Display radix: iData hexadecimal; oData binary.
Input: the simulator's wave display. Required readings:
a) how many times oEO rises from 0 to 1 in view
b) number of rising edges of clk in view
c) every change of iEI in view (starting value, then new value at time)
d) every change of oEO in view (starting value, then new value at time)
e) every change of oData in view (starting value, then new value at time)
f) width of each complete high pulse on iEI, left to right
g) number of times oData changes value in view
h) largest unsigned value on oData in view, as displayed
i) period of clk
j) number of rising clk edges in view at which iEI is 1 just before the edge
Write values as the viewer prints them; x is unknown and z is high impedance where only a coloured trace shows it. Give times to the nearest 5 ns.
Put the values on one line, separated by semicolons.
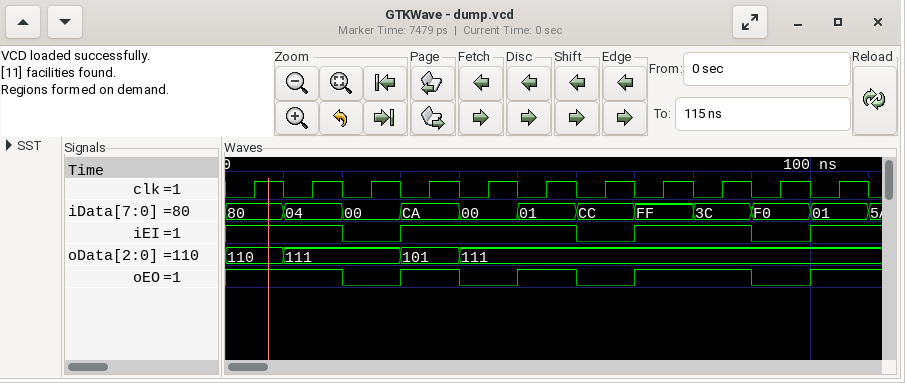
4; 11; 1, 0 at 20 ns, 1 at 30 ns, 0 at 60 ns, 1 at 70 ns, 0 at 90 ns, 1 at 100 ns; 1, 0 at 20 ns, 1 at 30 ns, 0 at 40 ns, 1 at 50 ns, 0 at 60 ns, 1 at 70 ns, 0 at 90 ns, 1 at 100 ns; 110, 111 at 10 ns, 101 at 30 ns, 111 at 40 ns; 30 ns, 20 ns; 3; 111; 10 ns; 8
